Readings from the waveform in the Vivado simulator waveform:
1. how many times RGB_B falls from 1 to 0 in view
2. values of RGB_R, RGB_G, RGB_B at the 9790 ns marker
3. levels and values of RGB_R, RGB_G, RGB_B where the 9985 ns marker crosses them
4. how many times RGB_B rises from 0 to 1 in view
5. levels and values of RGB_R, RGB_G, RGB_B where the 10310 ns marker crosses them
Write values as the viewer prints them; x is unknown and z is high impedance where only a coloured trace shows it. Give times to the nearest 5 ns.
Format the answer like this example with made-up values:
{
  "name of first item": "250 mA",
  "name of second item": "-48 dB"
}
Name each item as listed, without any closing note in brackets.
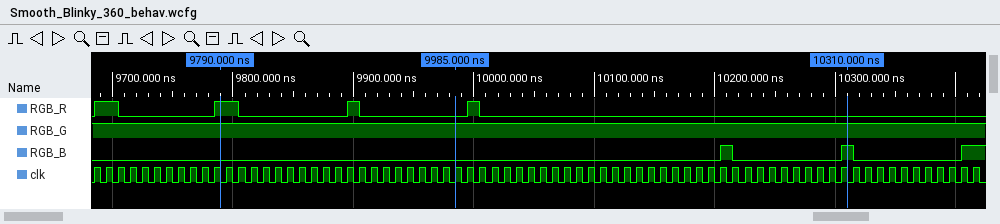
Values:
{
  "how many times RGB_B falls from 1 to 0 in view": "2",
  "values of RGB_R, RGB_G, RGB_B at the 9790 ns marker": "RGB_R=1, RGB_G=1, RGB_B=0",
  "levels and values of RGB_R, RGB_G, RGB_B where the 9985 ns marker crosses them": "RGB_R=0, RGB_G=1, RGB_B=0",
  "how many times RGB_B rises from 0 to 1 in view": "3",
  "levels and values of RGB_R, RGB_G, RGB_B where the 10310 ns marker crosses them": "RGB_R=0, RGB_G=1, RGB_B=1"
}
